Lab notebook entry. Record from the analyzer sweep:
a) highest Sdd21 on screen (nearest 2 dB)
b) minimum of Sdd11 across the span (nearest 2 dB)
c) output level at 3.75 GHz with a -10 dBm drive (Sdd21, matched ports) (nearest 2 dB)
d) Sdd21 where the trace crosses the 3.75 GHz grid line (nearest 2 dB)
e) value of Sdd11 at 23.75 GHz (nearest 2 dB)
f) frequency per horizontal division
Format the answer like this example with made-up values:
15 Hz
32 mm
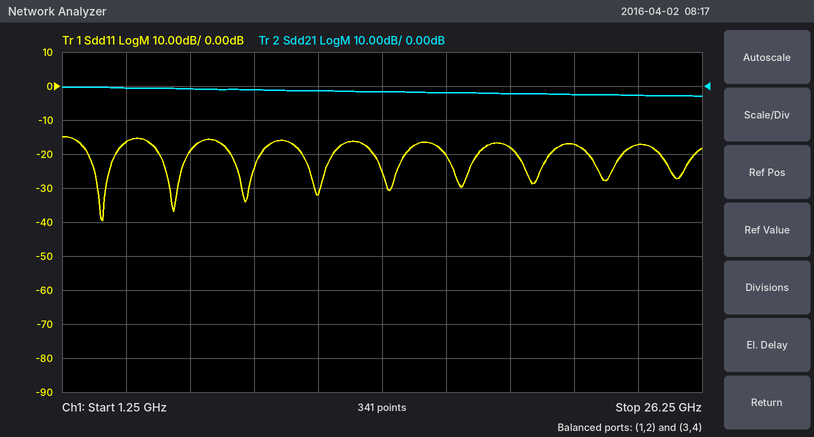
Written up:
0 dB
-40 dB
-10 dBm
0 dB
-18 dB
2.5 GHz
